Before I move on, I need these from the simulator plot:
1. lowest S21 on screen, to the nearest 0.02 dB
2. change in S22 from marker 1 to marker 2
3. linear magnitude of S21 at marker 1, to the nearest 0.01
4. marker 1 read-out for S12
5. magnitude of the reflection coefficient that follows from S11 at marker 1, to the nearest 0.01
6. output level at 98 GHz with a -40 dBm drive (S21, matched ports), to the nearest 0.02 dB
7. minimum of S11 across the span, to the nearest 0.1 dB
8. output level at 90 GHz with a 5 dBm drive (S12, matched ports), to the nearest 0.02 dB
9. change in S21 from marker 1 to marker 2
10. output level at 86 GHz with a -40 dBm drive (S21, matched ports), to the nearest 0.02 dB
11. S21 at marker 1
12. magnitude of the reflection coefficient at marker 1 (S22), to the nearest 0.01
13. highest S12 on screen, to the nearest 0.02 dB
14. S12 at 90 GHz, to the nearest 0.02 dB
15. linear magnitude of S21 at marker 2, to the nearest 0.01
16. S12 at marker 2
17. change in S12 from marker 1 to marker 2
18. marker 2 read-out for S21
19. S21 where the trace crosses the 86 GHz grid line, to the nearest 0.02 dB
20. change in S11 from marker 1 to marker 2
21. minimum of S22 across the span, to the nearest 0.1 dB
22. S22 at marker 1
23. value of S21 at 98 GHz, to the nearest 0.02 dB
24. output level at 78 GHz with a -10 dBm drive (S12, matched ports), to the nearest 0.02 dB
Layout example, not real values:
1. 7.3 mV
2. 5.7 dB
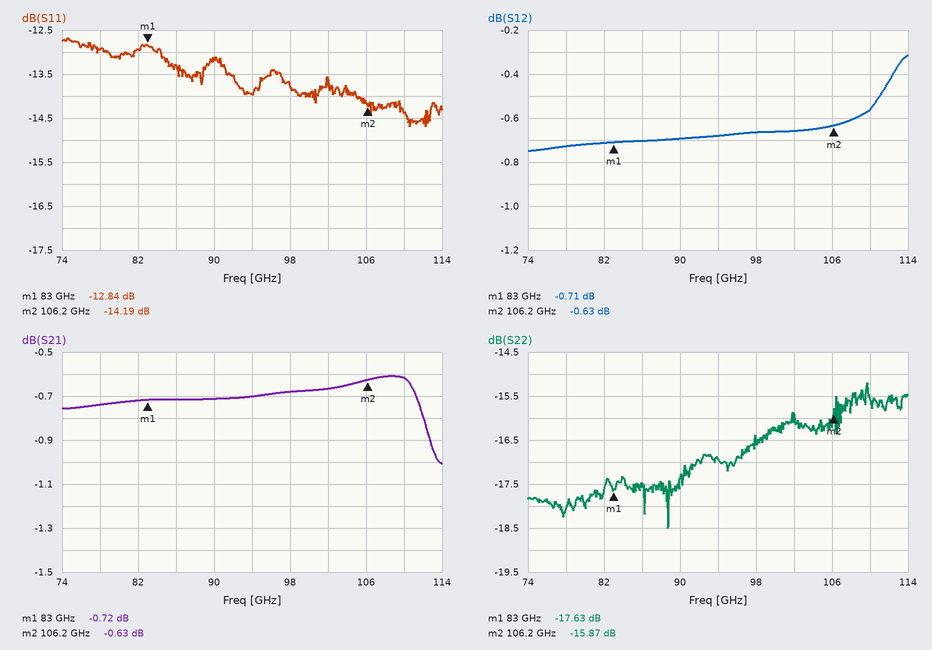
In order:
1. -1.00 dB
2. 1.76 dB
3. 0.92
4. -0.71 dB
5. 0.23
6. -40.68 dBm
7. -14.7 dB
8. 4.30 dBm
9. 0.09 dB
10. -40.72 dBm
11. -0.72 dB
12. 0.13
13. -0.32 dB
14. -0.70 dB
15. 0.93
16. -0.63 dB
17. 0.08 dB
18. -0.63 dB
19. -0.72 dB
20. -1.35 dB
21. -18.5 dB
22. -17.63 dB
23. -0.68 dB
24. -10.72 dBm
